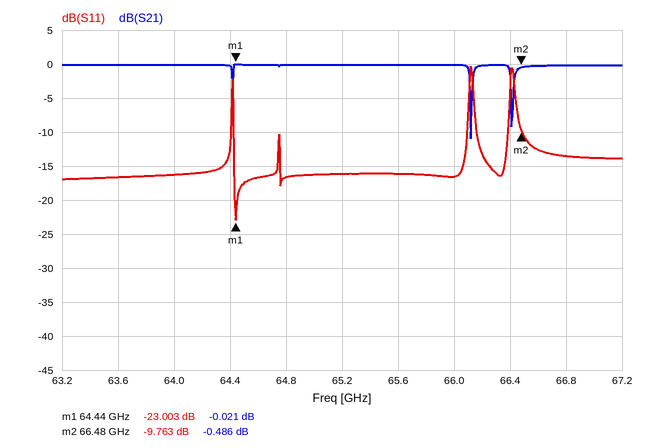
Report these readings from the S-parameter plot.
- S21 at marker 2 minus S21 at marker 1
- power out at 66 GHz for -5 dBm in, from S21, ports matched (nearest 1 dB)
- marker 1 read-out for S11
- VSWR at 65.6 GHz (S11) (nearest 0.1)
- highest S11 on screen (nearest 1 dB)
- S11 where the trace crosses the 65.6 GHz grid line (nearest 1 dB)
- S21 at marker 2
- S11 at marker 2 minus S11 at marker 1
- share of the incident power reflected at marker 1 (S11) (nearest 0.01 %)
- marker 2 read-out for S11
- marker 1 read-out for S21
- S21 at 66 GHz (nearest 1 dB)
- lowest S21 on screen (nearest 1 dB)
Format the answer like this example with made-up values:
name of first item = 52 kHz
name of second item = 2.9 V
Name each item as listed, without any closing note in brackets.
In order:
S21 at marker 2 minus S21 at marker 1 = -0.465 dB
power out at 66 GHz for -5 dBm in, from S21, ports matched = -5 dBm
marker 1 read-out for S11 = -23.003 dB
VSWR at 65.6 GHz (S11) = 1.4
highest S11 on screen = 0 dB
S11 where the trace crosses the 65.6 GHz grid line = -16 dB
S21 at marker 2 = -0.486 dB
S11 at marker 2 minus S11 at marker 1 = 13.240 dB
share of the incident power reflected at marker 1 (S11) = 0.50 %
marker 2 read-out for S11 = -9.763 dB
marker 1 read-out for S21 = -0.021 dB
S21 at 66 GHz = 0 dB
lowest S21 on screen = -11 dB
